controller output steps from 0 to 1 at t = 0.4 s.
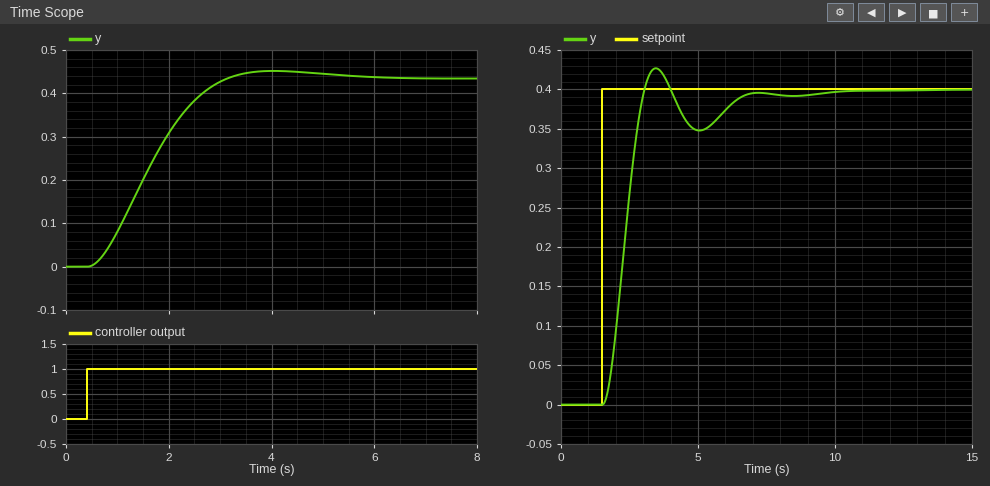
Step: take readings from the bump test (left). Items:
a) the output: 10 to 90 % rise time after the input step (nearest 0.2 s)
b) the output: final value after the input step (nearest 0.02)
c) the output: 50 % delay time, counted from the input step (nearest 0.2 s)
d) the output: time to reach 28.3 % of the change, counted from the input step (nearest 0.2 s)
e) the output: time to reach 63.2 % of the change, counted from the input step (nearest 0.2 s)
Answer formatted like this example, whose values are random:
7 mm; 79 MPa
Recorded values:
1.8 s; 0.44; 1.2 s; 0.8 s; 1.4 s
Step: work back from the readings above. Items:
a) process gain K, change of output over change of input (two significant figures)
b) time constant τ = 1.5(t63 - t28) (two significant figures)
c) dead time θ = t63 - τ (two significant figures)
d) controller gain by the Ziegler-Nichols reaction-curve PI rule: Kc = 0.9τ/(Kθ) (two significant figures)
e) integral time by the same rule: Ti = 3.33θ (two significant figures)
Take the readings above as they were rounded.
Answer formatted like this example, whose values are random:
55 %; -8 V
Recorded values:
0.44; 0.90 s; 0.50 s; 3.7; 1.7 s
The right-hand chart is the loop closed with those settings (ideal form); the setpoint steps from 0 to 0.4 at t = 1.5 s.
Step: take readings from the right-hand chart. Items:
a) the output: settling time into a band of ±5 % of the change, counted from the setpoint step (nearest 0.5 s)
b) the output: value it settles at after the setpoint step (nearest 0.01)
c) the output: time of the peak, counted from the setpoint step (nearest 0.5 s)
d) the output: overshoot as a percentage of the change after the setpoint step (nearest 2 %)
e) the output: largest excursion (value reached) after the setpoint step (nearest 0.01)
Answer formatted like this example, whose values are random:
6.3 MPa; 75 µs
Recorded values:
4.5 s; 0.40; 2.0 s; 6 %; 0.43
